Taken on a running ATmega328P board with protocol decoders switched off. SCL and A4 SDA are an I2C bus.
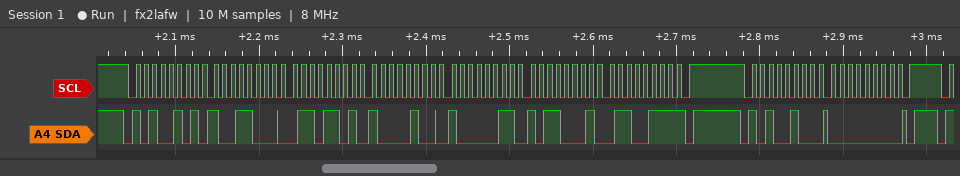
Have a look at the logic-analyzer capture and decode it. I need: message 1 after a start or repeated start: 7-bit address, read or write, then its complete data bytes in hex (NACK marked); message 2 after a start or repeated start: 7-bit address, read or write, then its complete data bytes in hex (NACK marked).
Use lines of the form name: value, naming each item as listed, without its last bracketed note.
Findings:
message 1 after a start or repeated start: 7-bit address, read or write, then its complete data bytes in hex: 0x52 read: 98 6D 84 83 B1 67 NACK
message 2 after a start or repeated start: 7-bit address, read or write, then its complete data bytes in hex: 0x52 write: 00
